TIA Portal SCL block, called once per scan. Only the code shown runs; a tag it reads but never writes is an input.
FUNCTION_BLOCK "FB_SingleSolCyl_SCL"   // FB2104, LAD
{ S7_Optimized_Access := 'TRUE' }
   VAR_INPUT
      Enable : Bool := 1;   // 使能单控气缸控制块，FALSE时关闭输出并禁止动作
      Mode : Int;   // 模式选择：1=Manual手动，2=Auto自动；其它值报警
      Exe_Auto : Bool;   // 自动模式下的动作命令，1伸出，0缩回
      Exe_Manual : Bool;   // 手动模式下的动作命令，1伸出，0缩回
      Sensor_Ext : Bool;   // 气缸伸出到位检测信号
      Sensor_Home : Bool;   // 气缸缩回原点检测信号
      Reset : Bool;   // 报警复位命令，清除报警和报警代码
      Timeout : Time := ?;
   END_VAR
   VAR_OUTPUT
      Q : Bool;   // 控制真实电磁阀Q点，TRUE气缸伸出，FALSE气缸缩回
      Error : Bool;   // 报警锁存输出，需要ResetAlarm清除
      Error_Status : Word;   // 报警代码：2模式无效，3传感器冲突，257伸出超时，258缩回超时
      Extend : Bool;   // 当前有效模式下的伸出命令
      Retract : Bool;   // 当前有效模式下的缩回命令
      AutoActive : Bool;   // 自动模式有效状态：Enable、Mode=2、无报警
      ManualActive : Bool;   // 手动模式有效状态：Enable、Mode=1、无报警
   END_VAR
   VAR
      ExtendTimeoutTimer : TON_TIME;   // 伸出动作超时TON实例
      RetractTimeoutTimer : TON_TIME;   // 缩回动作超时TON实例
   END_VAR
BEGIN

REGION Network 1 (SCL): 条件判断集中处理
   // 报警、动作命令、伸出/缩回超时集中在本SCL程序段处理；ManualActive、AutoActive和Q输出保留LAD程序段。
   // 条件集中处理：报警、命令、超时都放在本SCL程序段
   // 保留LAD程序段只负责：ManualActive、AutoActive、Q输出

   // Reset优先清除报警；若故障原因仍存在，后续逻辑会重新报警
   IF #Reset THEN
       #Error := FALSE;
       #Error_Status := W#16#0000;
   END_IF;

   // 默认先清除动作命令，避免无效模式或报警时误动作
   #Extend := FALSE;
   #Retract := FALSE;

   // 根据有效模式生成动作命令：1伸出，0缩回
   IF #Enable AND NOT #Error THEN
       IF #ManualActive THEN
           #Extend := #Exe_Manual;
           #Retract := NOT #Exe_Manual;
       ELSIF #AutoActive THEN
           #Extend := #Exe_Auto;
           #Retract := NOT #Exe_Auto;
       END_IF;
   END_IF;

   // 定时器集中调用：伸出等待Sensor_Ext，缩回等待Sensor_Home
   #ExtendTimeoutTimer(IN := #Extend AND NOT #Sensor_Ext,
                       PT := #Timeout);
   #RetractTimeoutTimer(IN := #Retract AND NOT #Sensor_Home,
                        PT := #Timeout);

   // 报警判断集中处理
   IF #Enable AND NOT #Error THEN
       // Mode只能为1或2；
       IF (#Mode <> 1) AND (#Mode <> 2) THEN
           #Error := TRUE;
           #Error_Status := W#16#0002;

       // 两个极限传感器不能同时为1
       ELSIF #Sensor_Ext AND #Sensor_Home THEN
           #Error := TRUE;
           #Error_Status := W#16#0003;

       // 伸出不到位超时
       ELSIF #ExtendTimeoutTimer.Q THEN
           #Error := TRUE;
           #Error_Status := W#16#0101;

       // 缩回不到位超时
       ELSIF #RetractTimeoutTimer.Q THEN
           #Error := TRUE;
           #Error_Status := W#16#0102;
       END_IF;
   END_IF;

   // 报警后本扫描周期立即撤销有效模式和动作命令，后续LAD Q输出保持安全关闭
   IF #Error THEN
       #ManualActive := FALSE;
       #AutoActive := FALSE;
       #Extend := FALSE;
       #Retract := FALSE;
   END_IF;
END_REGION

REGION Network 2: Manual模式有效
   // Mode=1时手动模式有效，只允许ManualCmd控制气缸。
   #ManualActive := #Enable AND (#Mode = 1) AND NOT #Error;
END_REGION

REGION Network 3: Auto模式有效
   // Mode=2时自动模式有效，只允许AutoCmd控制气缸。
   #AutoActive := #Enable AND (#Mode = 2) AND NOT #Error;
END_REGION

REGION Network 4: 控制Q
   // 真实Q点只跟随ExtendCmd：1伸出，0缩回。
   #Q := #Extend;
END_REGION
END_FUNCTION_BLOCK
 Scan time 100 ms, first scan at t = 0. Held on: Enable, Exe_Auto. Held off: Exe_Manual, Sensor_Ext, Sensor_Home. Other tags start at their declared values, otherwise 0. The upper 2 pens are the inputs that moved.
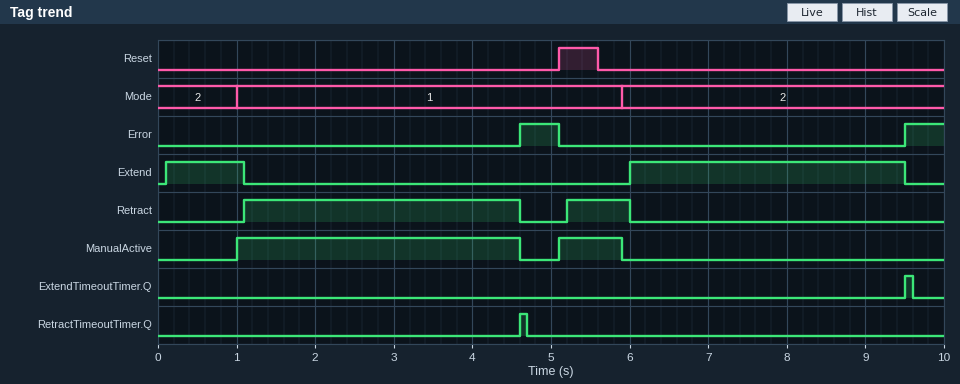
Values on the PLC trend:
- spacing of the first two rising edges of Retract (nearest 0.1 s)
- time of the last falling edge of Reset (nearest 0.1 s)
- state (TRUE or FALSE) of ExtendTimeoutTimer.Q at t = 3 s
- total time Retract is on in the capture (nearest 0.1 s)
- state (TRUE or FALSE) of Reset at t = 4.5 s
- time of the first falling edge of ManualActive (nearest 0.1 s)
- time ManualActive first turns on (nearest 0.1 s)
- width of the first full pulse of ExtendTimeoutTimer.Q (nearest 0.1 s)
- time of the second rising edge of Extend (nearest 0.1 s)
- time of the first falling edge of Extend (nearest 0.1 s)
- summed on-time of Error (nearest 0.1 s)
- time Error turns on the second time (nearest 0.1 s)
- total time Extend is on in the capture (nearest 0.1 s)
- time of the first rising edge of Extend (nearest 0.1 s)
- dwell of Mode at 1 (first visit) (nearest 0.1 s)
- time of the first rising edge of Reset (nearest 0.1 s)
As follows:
4.1 s
5.6 s
FALSE
4.3 s
FALSE
4.6 s
1.0 s
0.1 s
6.0 s
1.1 s
1.0 s
9.5 s
4.5 s
0.1 s
4.9 s
5.1 s
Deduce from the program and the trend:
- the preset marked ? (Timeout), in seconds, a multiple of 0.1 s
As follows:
3.5 s
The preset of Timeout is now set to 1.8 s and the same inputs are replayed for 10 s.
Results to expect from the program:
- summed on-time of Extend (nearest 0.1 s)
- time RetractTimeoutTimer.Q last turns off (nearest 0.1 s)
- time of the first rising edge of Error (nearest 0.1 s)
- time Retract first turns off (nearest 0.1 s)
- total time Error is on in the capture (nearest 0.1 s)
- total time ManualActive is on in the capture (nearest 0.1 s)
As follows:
2.8 s
3.0 s
2.9 s
2.9 s
4.4 s
2.7 s
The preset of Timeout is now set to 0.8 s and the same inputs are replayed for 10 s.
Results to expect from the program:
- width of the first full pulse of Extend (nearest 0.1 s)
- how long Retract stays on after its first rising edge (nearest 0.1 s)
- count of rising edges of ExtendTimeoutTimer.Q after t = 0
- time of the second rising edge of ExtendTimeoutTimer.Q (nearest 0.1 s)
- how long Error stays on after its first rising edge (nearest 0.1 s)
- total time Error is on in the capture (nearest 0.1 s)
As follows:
0.8 s
0.8 s
2
6.8 s
4.2 s
7.4 s
